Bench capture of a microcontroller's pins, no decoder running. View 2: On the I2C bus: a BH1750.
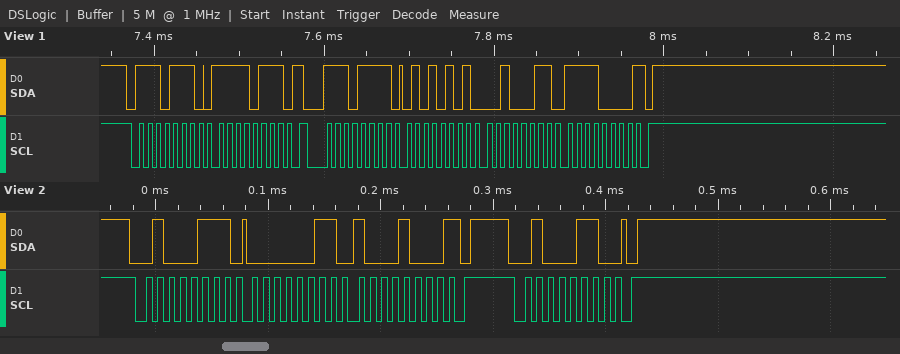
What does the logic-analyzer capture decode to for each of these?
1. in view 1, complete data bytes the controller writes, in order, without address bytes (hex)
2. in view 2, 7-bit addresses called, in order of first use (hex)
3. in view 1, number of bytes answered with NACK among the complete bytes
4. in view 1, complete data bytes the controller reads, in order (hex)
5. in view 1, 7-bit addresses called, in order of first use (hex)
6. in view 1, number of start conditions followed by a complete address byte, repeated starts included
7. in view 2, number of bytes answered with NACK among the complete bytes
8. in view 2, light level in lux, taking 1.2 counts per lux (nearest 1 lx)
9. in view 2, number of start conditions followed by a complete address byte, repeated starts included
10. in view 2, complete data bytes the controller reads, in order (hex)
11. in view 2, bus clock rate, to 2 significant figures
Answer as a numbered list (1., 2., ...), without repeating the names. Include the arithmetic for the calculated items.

1. F7
2. 0x23
3. 1
4. 55 23 F0
5. 0x77
6. 2
7. 1
8. 904 / 1.2 = 753 lx
9. 2
10. 03 88
11. 100 kHz
